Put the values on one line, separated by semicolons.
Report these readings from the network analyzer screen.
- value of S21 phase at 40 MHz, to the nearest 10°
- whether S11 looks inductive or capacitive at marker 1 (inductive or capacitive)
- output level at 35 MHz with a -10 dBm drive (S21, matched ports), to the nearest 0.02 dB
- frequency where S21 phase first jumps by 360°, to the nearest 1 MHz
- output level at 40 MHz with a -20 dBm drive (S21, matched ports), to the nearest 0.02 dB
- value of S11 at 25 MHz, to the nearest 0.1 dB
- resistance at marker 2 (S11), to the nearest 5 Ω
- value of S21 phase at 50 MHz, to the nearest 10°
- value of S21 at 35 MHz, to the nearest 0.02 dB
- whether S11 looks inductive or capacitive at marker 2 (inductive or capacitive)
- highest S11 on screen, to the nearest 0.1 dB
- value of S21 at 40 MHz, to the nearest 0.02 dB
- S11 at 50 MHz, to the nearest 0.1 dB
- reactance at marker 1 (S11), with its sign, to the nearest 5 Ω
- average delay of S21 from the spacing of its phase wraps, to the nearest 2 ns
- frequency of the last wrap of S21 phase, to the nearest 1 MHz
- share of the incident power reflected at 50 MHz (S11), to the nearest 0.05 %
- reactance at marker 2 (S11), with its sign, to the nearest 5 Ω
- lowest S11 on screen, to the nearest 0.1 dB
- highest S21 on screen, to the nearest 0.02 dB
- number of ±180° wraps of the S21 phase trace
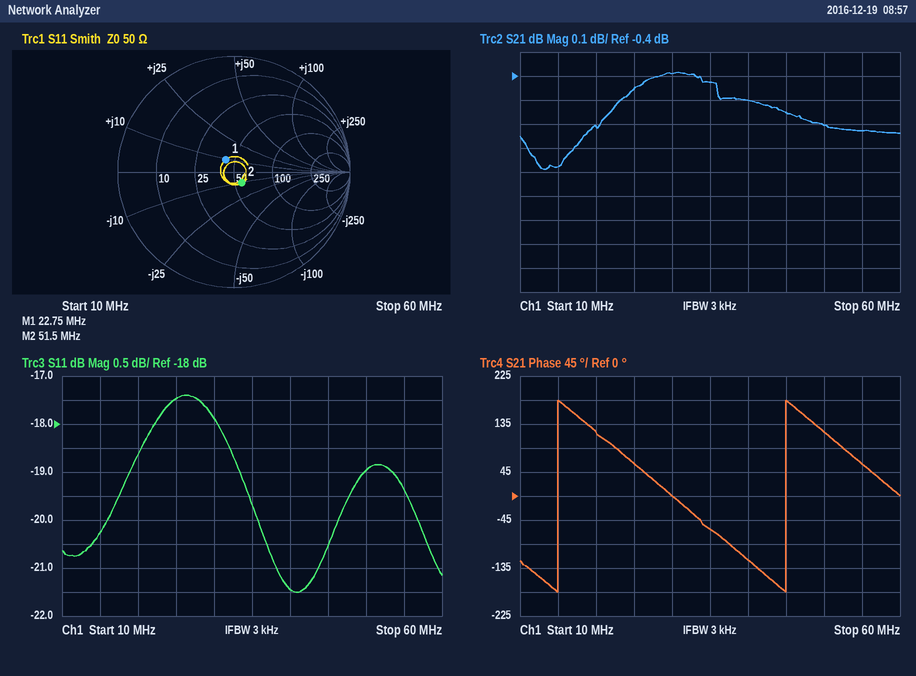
-120°; inductive; -10.42 dBm; 15 MHz; -20.50 dBm; -17.5 dB; 55 Ω; 120°; -0.42 dB; capacitive; -17.4 dB; -0.50 dB; -19.0 dB; +10 Ω; 34 ns; 45 MHz; 1.25 %; -10 Ω; -21.5 dB; -0.38 dB; 2
